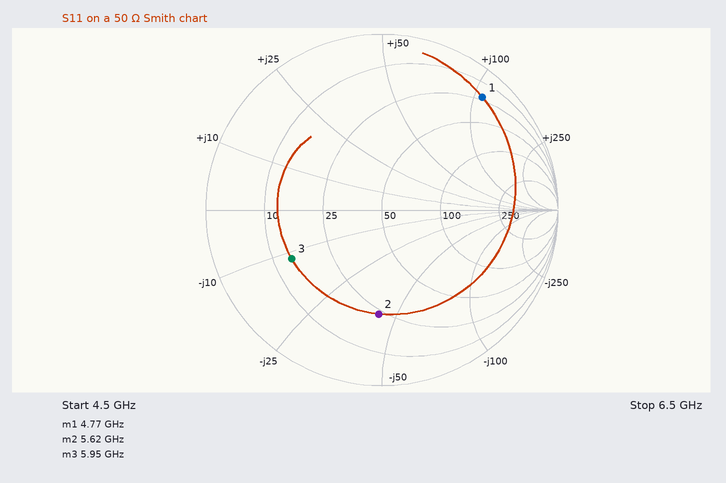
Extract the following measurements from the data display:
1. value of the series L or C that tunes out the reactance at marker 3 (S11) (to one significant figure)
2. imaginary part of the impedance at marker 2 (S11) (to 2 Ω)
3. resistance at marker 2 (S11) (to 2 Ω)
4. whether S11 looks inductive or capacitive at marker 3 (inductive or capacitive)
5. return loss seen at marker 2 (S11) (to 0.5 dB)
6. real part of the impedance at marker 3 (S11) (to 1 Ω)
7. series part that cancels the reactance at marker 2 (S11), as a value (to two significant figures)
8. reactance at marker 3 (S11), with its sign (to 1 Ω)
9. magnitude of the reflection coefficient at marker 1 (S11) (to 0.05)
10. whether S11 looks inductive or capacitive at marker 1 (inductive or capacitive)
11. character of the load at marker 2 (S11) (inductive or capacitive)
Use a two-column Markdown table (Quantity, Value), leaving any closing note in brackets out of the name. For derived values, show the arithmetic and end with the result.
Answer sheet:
| Quantity | Value |
|---|---|
| value of the series L or C that tunes out the reactance at marker 3 (S11) | L = 12 Ω/(2π × 5.95 GHz) ≈ 321 pH, so 300 pH to one significant figure |
| imaginary part of the impedance at marker 2 (S11) | -42 Ω |
| resistance at marker 2 (S11) | 24 Ω |
| whether S11 looks inductive or capacitive at marker 3 | capacitive |
| return loss seen at marker 2 (S11) | 4.5 dB |
| real part of the impedance at marker 3 (S11) | 14 Ω |
| series part that cancels the reactance at marker 2 (S11), as a value | L = 42 Ω/(2π × 5.62 GHz) ≈ 1.2 nH |
| reactance at marker 3 (S11), with its sign | -12 Ω |
| magnitude of the reflection coefficient at marker 1 (S11) | 0.85 |
| whether S11 looks inductive or capacitive at marker 1 | inductive |
| character of the load at marker 2 (S11) | capacitive |
